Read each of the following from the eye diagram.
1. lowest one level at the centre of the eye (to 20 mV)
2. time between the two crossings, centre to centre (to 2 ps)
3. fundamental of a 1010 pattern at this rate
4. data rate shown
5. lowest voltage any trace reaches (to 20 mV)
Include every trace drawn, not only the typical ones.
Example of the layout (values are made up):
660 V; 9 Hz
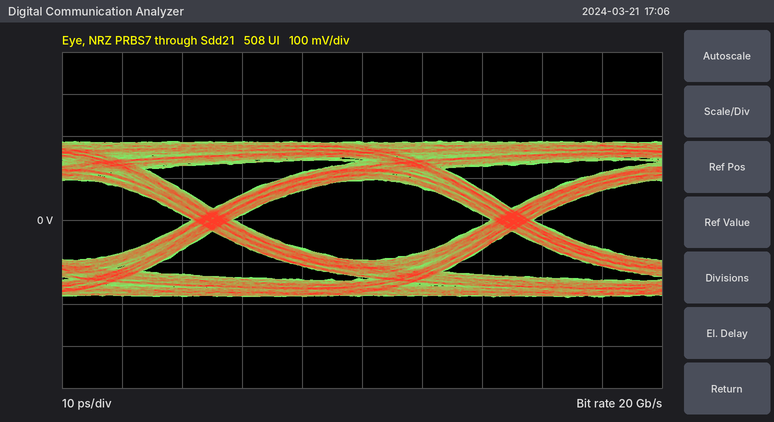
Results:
100 mV; 50 ps; 10 GHz; 20 Gb/s; -180 mV
